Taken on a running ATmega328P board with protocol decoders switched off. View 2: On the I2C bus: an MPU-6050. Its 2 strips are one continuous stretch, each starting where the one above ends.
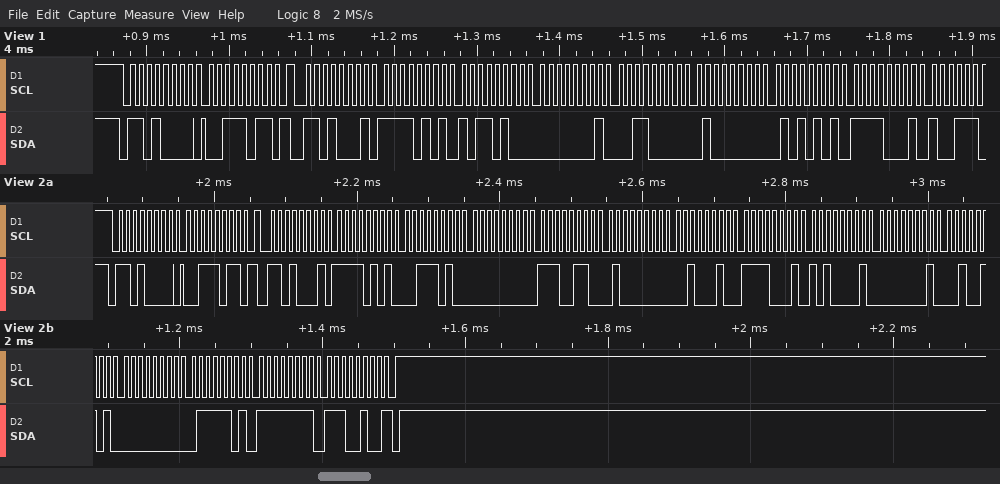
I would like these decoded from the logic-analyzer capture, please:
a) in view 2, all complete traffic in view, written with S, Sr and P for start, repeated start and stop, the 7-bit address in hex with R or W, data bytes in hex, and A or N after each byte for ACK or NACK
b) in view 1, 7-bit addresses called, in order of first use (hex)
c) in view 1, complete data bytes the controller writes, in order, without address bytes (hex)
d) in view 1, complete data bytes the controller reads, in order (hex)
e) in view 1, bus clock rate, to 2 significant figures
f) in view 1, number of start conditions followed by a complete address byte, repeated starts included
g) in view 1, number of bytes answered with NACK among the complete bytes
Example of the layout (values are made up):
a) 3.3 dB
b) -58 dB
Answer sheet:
a) S 68W A 3B A Sr 68R A F5 A 3A A 00 A E6 A 40 A 22 A F1 A A1 A 01 A 25 A 00 A 7D A FF A E4 N P
b) 0x68
c) 3B
d) F5 B4 01 30 40 55 F1
e) 100 kHz
f) 2
g) 0
